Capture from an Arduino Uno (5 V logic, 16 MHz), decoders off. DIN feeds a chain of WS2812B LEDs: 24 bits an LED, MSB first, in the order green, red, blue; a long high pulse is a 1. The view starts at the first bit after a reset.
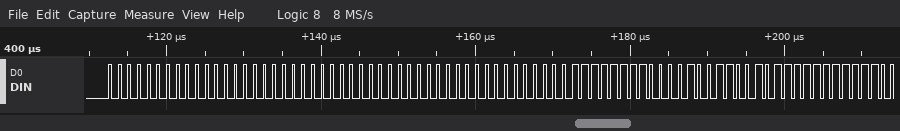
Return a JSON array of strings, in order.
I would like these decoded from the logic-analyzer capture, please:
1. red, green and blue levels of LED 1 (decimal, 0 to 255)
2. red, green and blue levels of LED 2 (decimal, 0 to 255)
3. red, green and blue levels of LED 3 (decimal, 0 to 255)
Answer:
["0, 0, 0", "0, 0, 0", "9, 255, 151"]
